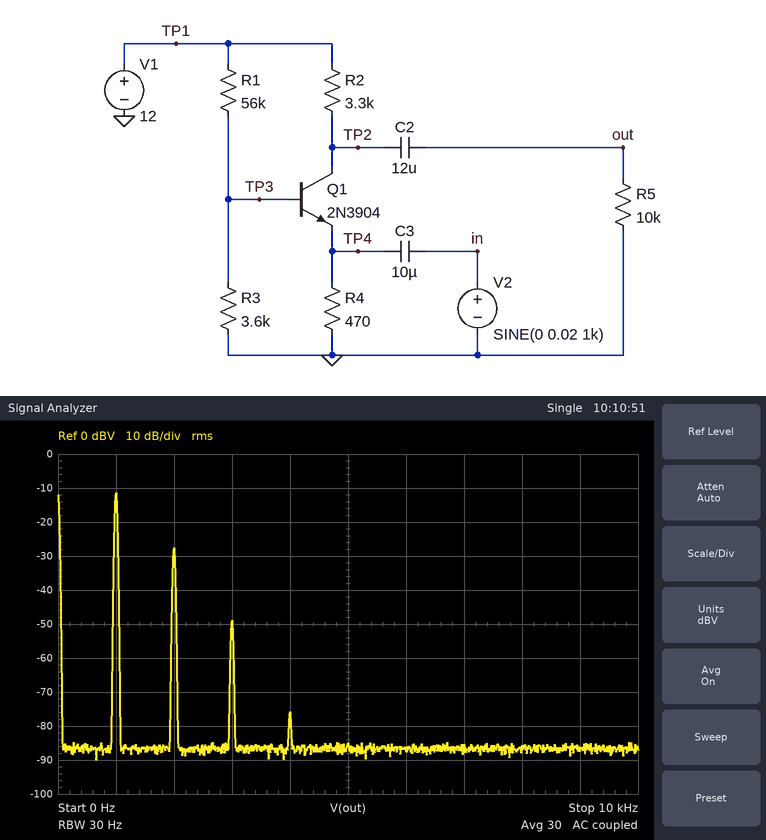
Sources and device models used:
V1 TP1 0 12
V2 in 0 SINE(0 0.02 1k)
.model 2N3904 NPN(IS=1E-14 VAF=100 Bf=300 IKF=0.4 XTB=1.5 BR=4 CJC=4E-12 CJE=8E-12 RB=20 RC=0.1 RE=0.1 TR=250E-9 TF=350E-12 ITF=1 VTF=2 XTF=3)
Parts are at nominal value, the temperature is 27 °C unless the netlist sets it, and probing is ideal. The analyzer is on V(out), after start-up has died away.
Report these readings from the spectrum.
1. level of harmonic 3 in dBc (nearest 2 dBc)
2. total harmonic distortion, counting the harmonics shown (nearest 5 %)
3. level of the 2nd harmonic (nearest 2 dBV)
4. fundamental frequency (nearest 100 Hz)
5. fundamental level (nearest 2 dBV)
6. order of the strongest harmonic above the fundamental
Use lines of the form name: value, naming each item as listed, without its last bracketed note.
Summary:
level of harmonic 3 in dBc: -38 dBc
total harmonic distortion, counting the harmonics shown: 15 %
level of the 2nd harmonic: -28 dBV
fundamental frequency: 1.0 kHz
fundamental level: -12 dBV
order of the strongest harmonic above the fundamental: 2
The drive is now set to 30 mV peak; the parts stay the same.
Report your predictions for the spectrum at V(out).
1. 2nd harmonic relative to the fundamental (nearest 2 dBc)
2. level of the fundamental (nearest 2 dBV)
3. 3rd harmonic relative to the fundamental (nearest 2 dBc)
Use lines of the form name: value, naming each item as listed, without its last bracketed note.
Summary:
2nd harmonic relative to the fundamental: -12 dBc
level of the fundamental: -8 dBV
3rd harmonic relative to the fundamental: -30 dBc
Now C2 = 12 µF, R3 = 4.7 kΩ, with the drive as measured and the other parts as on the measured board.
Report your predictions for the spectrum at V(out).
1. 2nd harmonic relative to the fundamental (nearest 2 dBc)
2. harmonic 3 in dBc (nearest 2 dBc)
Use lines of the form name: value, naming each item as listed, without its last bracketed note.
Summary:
2nd harmonic relative to the fundamental: -20 dBc
harmonic 3 in dBc: -50 dBc
